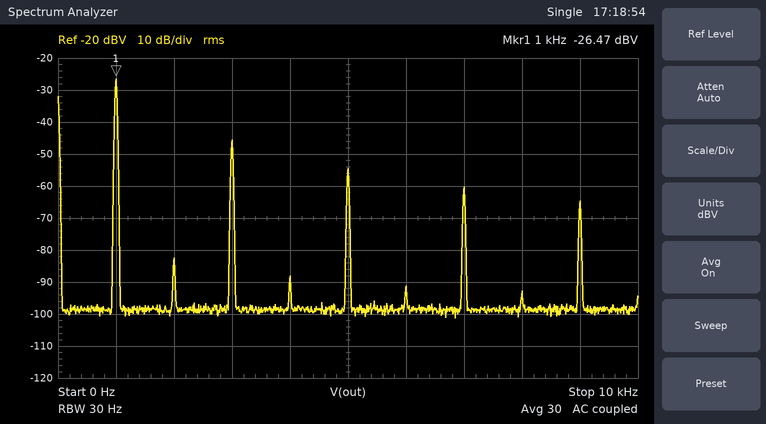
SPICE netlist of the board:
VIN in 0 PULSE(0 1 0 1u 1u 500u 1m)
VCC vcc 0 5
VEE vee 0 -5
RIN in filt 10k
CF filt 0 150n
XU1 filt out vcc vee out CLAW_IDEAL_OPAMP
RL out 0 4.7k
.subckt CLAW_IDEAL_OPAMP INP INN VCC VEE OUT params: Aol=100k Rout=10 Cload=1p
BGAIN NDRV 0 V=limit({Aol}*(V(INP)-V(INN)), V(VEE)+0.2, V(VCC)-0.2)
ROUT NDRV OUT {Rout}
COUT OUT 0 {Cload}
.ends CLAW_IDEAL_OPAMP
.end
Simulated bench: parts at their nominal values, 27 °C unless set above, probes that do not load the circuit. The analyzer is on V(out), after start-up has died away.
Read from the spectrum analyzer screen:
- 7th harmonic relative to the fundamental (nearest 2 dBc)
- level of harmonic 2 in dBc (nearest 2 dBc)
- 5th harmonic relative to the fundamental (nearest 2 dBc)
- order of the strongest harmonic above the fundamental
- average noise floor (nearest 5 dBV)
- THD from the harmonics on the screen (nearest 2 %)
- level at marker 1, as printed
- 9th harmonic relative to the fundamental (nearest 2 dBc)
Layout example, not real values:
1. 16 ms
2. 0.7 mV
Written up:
1. -34 dBc
2. -56 dBc
3. -28 dBc
4. 3
5. -100 dBV
6. 12 %
7. -26.47 dBV
8. -38 dBc
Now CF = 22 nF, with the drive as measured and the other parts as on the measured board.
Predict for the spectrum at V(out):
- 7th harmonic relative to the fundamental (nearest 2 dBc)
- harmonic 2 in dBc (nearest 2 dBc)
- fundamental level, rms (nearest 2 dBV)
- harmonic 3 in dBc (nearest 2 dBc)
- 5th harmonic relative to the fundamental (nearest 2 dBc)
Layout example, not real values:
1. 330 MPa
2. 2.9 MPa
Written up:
1. -32 dBc
2. -54 dBc
3. -12 dBV
4. -18 dBc
5. -26 dBc
